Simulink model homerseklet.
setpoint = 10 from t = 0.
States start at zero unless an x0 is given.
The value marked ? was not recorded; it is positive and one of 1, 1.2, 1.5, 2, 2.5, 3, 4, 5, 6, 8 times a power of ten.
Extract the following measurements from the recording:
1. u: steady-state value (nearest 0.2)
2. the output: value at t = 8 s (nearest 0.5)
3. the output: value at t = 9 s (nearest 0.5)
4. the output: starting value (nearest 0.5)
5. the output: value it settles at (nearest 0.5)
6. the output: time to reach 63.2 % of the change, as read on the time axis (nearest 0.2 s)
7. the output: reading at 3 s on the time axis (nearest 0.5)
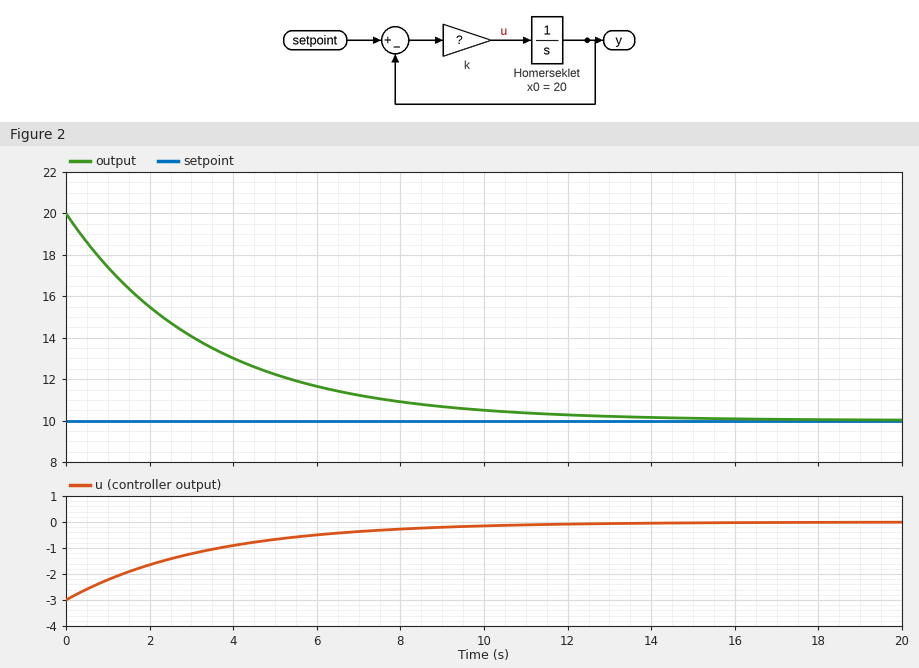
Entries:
0.0
11.0
10.5
20.0
10.0
3.4 s
14.0
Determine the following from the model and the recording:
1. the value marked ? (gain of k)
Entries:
0.3
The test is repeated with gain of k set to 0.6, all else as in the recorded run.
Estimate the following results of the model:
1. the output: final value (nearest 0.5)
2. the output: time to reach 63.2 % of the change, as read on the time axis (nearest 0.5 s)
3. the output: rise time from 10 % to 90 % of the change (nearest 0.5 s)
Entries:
10.0
1.5 s
3.5 s
